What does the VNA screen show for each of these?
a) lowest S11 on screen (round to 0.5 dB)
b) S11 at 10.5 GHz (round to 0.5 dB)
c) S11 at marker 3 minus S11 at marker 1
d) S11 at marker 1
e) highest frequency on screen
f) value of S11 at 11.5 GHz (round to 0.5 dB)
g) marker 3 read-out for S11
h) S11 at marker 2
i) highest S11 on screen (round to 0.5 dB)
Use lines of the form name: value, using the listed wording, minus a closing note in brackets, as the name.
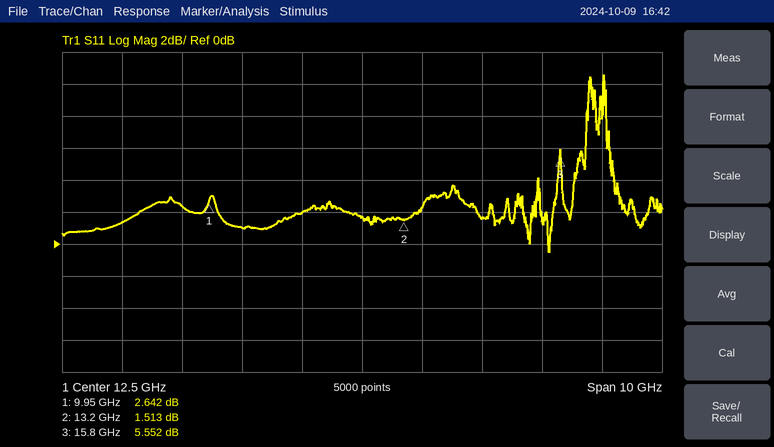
lowest S11 on screen: -0.5 dB
S11 at 10.5 GHz: 1.0 dB
S11 at marker 3 minus S11 at marker 1: 2.910 dB
S11 at marker 1: 2.642 dB
highest frequency on screen: 17.5 GHz
value of S11 at 11.5 GHz: 2.0 dB
marker 3 read-out for S11: 5.552 dB
S11 at marker 2: 1.513 dB
highest S11 on screen: 10.5 dB
